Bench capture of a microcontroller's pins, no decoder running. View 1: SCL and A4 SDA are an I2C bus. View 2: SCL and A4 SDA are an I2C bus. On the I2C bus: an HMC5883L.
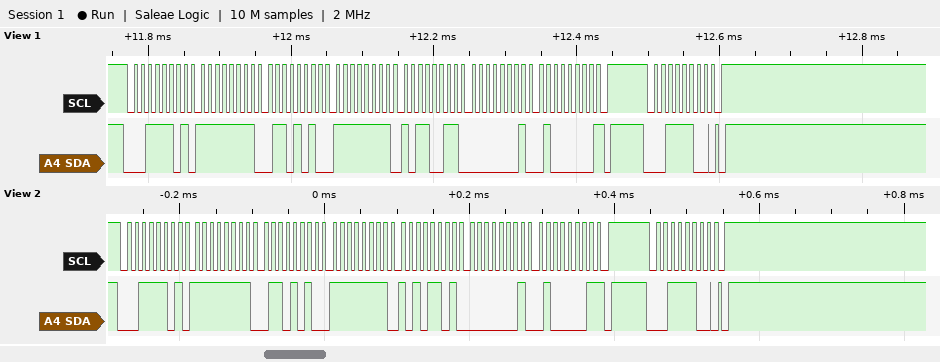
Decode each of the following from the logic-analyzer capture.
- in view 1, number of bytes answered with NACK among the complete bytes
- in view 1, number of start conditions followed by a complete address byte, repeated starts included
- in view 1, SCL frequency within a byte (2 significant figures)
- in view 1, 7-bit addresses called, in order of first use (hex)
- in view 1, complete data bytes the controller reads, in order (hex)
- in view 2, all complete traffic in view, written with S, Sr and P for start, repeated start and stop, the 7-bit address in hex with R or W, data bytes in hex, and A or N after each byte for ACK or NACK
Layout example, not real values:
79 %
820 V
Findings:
1
2
100 kHz
0x1E
FF 6A FF B3 01 40
S 1ER A FF A 6A A FF A AD A 01 A 41 N P S 1EW A P
